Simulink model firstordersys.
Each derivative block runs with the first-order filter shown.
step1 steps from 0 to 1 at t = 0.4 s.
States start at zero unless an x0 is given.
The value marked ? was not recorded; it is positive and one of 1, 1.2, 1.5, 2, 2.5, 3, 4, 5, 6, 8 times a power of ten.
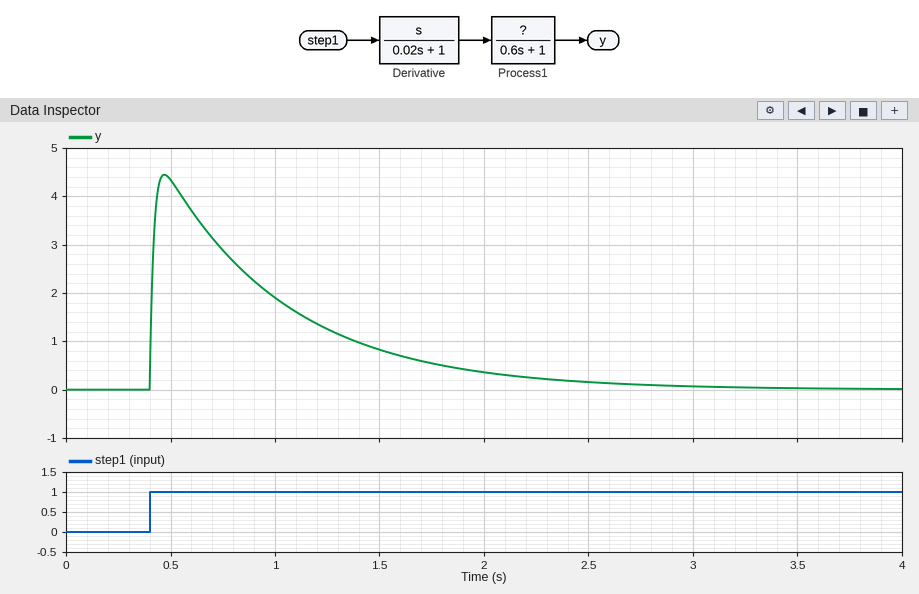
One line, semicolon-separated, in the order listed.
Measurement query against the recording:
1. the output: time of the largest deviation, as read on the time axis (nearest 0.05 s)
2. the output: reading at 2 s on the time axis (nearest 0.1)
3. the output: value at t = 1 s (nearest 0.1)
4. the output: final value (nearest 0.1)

0.45 s; 0.4; 1.9; 0.0
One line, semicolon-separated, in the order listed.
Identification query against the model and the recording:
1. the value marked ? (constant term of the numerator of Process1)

3
